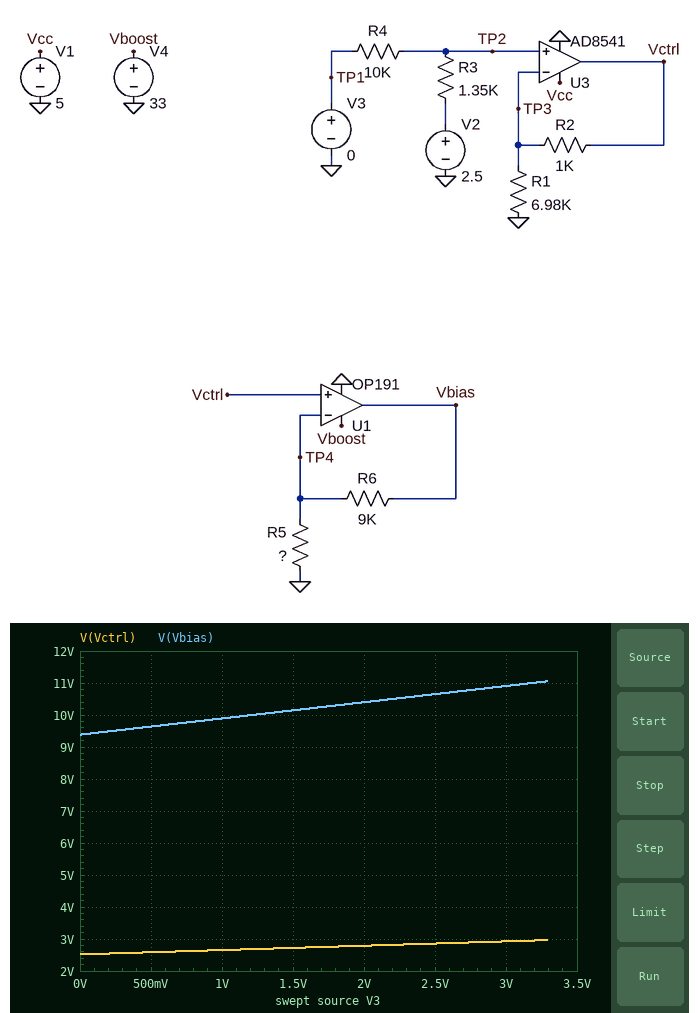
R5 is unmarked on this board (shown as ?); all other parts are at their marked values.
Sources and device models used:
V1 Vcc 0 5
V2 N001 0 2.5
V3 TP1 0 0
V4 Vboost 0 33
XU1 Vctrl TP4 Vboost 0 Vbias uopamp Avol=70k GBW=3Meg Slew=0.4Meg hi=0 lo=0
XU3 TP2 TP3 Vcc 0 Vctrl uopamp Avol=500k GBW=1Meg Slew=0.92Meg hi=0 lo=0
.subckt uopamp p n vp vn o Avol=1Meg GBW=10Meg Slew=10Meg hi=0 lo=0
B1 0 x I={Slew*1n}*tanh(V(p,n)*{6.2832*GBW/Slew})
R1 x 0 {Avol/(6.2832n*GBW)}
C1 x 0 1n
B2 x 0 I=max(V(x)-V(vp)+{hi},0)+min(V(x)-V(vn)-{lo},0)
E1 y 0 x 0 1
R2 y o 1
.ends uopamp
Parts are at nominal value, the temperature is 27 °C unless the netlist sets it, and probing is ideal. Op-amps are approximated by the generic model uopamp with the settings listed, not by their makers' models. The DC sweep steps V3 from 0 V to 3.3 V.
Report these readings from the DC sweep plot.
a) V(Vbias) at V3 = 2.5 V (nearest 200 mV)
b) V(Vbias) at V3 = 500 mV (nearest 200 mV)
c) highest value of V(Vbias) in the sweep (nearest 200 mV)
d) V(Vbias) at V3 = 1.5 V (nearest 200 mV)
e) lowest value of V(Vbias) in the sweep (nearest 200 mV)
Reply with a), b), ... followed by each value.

a) 10.6 V
b) 9.6 V
c) 11.0 V
d) 10.2 V
e) 9.4 V
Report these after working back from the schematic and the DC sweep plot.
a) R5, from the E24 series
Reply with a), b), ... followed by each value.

a) 3.3 kΩ
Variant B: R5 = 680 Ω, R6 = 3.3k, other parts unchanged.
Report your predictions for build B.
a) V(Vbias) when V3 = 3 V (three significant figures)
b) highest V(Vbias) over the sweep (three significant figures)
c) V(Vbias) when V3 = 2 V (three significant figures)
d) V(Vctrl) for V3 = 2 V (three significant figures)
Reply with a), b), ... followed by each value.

a) 17.1 V
b) 17.4 V
c) 16.3 V
d) 2.79 V
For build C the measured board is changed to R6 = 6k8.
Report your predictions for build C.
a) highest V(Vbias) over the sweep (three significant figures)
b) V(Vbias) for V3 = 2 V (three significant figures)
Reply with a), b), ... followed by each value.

a) 9.08 V
b) 8.54 V
